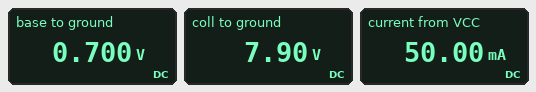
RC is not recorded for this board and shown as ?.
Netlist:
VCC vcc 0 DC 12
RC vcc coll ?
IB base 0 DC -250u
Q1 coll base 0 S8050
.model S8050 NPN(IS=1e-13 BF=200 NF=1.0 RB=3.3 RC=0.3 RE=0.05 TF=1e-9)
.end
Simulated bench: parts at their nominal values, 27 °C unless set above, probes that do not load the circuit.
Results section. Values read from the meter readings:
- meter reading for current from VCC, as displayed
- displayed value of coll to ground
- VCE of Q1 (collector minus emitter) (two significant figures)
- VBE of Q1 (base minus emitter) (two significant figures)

50.00 mA
7.90 V
7.9 V
700 mV
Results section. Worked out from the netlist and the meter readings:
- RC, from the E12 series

82 Ω
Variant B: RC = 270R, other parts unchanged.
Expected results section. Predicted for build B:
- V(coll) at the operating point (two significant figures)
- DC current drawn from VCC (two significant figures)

200 mV
44 mA
